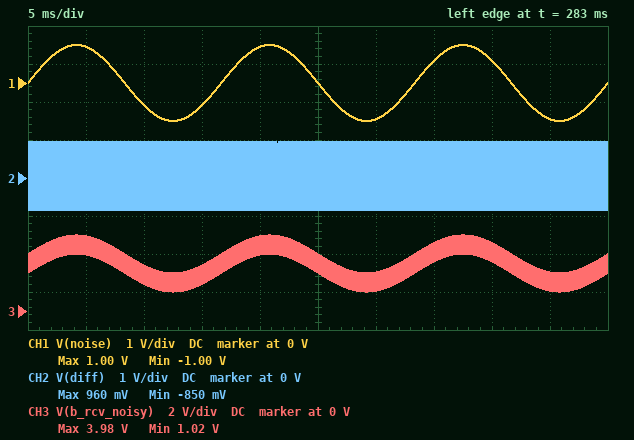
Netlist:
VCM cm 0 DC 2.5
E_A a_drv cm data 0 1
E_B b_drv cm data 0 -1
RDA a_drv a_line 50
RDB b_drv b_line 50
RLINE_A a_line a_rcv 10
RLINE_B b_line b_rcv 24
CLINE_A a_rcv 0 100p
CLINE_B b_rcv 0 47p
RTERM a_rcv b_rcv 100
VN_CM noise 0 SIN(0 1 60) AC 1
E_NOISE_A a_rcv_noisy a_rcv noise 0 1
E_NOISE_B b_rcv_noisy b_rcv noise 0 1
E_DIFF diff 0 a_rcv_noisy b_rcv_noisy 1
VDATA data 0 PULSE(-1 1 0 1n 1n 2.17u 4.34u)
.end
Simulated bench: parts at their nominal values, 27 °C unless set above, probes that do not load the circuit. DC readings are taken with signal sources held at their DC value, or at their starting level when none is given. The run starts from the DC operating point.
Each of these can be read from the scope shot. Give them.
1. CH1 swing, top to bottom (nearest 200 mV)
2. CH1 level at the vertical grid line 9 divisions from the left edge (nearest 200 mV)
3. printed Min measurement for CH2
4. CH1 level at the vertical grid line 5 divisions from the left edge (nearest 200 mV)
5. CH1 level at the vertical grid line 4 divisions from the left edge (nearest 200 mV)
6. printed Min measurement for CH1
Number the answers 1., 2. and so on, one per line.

1. 2.0 V
2. -1.0 V
3. -850 mV
4. 0 V
5. 1.0 V
6. -1.00 V
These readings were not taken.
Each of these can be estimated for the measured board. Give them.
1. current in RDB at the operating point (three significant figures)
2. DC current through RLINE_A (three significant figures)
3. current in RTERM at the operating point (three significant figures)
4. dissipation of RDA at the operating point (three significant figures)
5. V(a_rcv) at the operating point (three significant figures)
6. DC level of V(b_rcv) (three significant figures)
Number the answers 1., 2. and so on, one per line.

1. 8.55 mA
2. 8.55 mA
3. 8.55 mA
4. 3.65 mW
5. 2.01 V
6. 2.87 V
